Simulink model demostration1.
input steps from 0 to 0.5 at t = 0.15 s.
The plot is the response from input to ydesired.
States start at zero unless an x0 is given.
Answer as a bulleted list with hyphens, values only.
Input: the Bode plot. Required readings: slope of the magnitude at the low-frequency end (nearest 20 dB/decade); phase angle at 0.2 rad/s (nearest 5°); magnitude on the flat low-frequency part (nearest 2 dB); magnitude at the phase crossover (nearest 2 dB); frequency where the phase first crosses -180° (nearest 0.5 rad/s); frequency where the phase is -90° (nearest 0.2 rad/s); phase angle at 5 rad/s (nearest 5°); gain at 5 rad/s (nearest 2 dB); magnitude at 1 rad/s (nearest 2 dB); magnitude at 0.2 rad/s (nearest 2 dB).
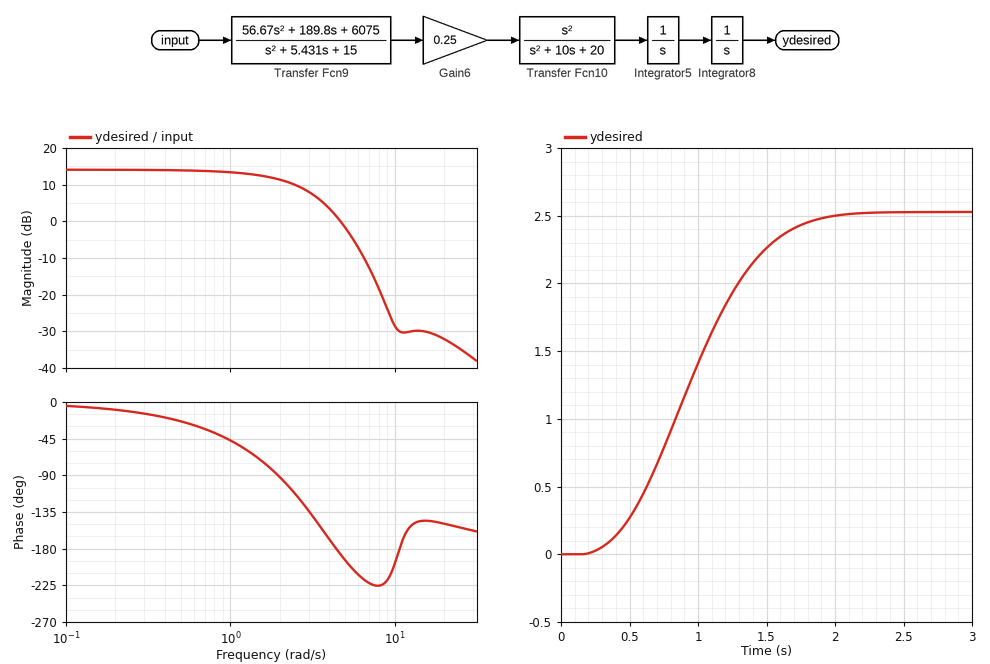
- 0 dB/decade
- -10°
- 14 dB
- 2 dB
- 4.5 rad/s
- 2.0 rad/s
- -195°
- -2 dB
- 14 dB
- 14 dB
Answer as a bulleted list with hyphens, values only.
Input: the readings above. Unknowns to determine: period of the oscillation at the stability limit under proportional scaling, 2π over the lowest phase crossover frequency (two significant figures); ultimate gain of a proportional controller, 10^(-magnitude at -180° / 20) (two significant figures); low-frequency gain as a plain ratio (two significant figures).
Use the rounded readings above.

- 1.4 s
- 0.79
- 5.0
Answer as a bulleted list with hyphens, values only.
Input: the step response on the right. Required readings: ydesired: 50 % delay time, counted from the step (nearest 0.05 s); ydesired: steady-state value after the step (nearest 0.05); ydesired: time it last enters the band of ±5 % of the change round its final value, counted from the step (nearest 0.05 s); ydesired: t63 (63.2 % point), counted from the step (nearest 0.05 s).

- 0.80 s
- 2.55
- 1.55 s
- 0.95 s
